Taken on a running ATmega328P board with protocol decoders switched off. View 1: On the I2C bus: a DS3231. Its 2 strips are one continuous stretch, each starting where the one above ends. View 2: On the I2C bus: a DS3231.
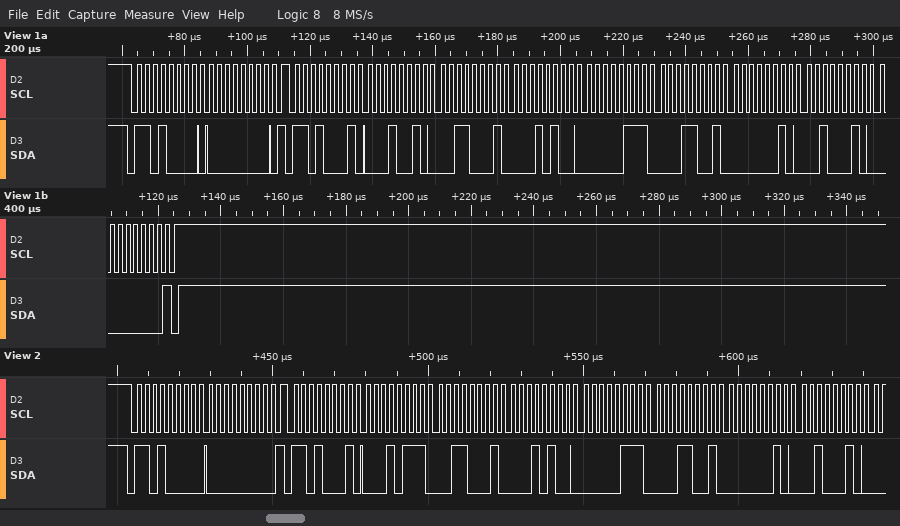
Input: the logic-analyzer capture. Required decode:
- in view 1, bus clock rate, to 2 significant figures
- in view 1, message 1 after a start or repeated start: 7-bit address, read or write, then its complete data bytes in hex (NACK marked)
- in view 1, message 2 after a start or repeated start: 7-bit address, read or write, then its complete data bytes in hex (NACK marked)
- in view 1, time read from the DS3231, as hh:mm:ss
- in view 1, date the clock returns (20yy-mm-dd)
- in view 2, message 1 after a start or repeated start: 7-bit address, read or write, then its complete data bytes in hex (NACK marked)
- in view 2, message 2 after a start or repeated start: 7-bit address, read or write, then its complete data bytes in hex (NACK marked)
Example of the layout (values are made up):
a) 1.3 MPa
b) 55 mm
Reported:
a) 400 kHz
b) 0x68 write: 00
c) 0x68 read: 12 31 14 07 19 02 22 00 NACK
d) 14:31:12
e) 2022-02-19
f) 0x68 write: 00
g) 0x68 read: 17 31 14 07 19 02 22
